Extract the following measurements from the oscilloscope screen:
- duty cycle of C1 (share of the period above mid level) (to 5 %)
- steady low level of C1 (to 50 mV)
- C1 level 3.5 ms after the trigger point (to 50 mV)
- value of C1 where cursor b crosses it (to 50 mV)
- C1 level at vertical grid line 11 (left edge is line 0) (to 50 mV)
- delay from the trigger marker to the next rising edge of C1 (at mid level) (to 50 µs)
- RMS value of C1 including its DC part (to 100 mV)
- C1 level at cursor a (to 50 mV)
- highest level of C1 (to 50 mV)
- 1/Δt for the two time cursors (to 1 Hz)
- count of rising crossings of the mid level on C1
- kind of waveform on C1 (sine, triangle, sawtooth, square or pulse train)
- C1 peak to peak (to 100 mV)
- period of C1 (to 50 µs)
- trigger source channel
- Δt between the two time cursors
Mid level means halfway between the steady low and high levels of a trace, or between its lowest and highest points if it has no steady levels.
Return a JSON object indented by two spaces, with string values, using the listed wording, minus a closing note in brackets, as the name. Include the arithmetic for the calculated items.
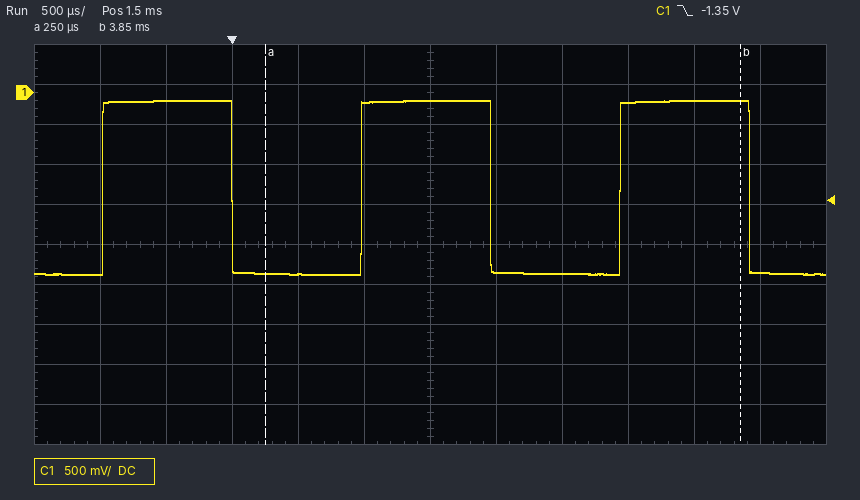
{
  "duty cycle of C1 (share of the period above mid level)": "50 %",
  "steady low level of C1": "-2.25 V",
  "C1 level 3.5 ms after the trigger point": "-100 mV",
  "value of C1 where cursor b crosses it": "-100 mV",
  "C1 level at vertical grid line 11 (left edge is line 0)": "-2.25 V",
  "delay from the trigger marker to the next rising edge of C1 (at mid level)": "1.00 ms",
  "RMS value of C1 including its DC part": "√(0.5 × (-100 mV)² + 0.5 × (-2.25 V)²) ≈ 1.6 V",
  "C1 level at cursor a": "-2.25 V",
  "highest level of C1": "-100 mV",
  "1/Δt for the two time cursors": "1 / 3.60 ms ≈ 278 Hz",
  "count of rising crossings of the mid level on C1": "3",
  "kind of waveform on C1": "square",
  "C1 peak to peak": "2.20 V",
  "period of C1": "1.95 ms",
  "trigger source channel": "C1",
  "Δt between the two time cursors": "3.85 ms − (250 µs) = 3.60 ms"
}
